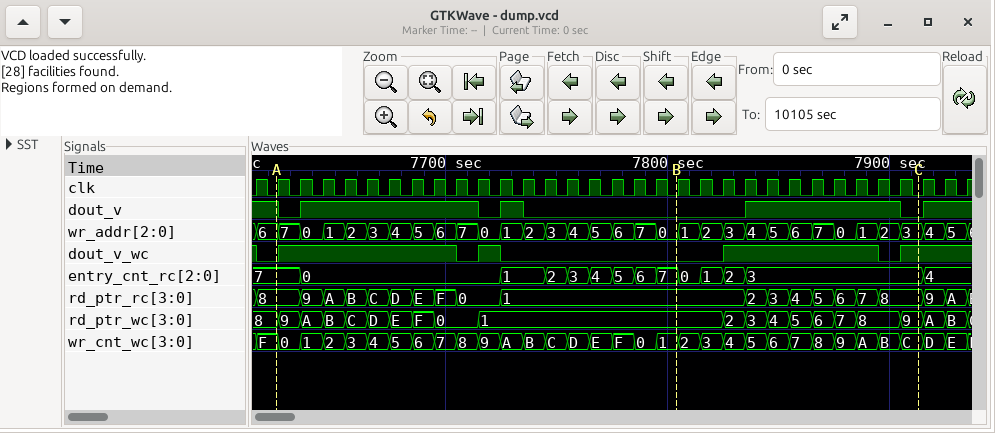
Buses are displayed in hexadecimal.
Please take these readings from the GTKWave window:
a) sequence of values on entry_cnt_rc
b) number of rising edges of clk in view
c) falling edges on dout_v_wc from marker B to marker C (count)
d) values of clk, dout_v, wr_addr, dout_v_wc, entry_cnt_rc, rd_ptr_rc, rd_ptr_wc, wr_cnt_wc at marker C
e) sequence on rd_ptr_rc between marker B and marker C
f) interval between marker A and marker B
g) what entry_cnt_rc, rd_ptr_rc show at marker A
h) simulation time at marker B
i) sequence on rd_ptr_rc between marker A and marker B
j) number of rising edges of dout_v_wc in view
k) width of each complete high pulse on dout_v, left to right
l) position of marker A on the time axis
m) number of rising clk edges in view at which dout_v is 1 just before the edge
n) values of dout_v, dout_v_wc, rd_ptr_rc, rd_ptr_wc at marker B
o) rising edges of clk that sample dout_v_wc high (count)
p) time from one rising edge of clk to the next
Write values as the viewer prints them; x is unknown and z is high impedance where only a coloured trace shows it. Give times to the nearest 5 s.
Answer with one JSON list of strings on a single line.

["7, 0, 1, 2, 3, 4, 5, 6, 7, 0, 1, 2, 3, 4", "33", "1", "clk=0, dout_v=0, wr_addr=3, dout_v_wc=1, entry_cnt_rc=3, rd_ptr_rc=8, rd_ptr_wc=9, wr_cnt_wc=C", "1, 2, 3, 4, 5, 6, 7, 8", "180 s", "entry_cnt_rc=7, rd_ptr_rc=8", "7805 s", "8, 9, A, B, C, D, E, F, 0, 1", "4", "80 s, 10 s, 70 s", "7625 s", "20", "dout_v=0, dout_v_wc=0, rd_ptr_rc=1, rd_ptr_wc=1", "20", "10 s"]
